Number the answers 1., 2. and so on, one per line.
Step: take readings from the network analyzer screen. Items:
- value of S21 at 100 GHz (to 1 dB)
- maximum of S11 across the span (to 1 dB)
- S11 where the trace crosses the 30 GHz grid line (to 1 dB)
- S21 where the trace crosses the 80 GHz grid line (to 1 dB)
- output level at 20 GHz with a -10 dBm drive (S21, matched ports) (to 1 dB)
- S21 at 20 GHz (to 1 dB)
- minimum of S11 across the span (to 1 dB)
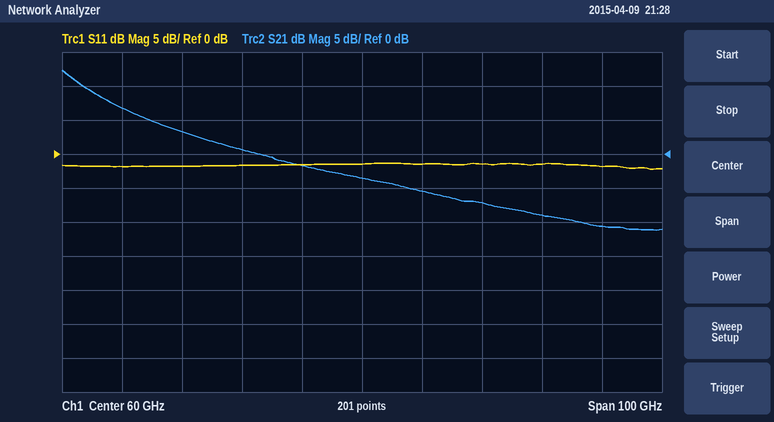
1. -11 dB
2. -1 dB
3. -2 dB
4. -7 dB
5. -3 dBm
6. 7 dB
7. -2 dB
